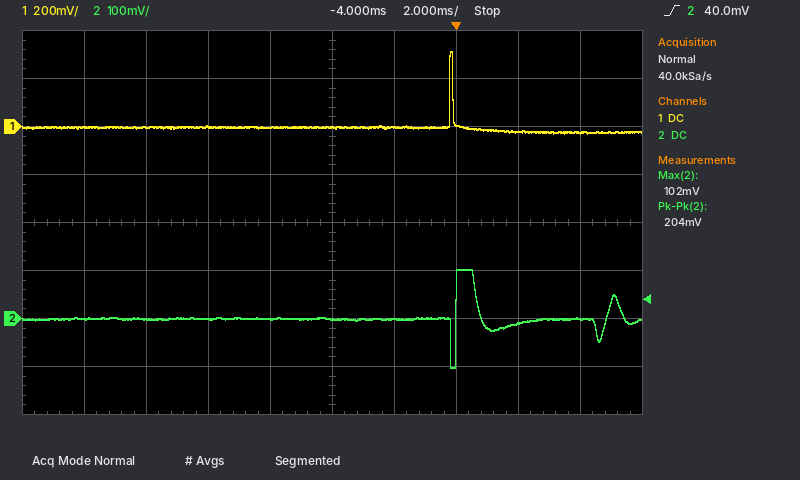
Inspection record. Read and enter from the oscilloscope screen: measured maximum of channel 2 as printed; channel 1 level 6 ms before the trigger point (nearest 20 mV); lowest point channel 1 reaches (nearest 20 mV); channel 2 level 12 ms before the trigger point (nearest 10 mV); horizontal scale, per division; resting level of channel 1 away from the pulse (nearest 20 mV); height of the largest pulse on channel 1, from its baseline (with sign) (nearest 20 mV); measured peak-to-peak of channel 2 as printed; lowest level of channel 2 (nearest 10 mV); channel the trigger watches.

102 mV
0 mV
-20 mV
0 mV
2 ms
0 mV
+320 mV
204 mV
-100 mV
channel 2
